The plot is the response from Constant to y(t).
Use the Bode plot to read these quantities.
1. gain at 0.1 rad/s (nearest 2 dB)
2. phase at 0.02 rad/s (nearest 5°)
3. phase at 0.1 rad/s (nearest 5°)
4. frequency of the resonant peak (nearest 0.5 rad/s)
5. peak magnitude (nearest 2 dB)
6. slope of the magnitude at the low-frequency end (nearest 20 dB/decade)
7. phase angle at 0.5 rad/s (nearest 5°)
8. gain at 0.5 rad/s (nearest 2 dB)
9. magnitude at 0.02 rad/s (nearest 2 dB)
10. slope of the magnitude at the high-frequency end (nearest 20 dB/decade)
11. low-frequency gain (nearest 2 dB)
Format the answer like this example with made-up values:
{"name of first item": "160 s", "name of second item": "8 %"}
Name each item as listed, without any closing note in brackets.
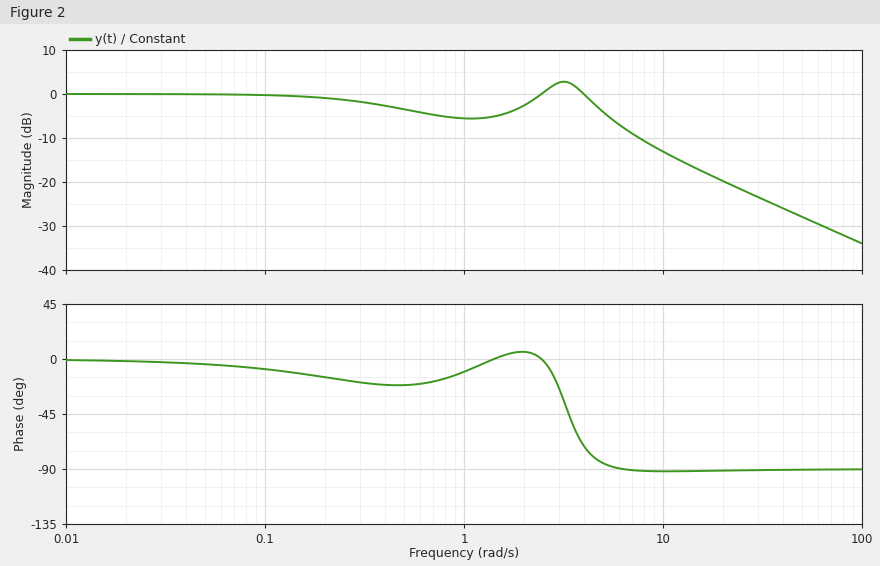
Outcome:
{"gain at 0.1 rad/s": "0 dB", "phase at 0.02 rad/s": "0°", "phase at 0.1 rad/s": "-10°", "frequency of the resonant peak": "3.0 rad/s", "peak magnitude": "2 dB", "slope of the magnitude at the low-frequency end": "0 dB/decade", "phase angle at 0.5 rad/s": "-20°", "gain at 0.5 rad/s": "-4 dB", "magnitude at 0.02 rad/s": "0 dB", "slope of the magnitude at the high-frequency end": "-20 dB/decade", "low-frequency gain": "0 dB"}
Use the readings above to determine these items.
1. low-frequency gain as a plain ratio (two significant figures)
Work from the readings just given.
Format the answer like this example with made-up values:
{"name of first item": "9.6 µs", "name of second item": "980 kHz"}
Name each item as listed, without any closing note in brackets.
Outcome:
{"low-frequency gain as a plain ratio": "1.0"}
